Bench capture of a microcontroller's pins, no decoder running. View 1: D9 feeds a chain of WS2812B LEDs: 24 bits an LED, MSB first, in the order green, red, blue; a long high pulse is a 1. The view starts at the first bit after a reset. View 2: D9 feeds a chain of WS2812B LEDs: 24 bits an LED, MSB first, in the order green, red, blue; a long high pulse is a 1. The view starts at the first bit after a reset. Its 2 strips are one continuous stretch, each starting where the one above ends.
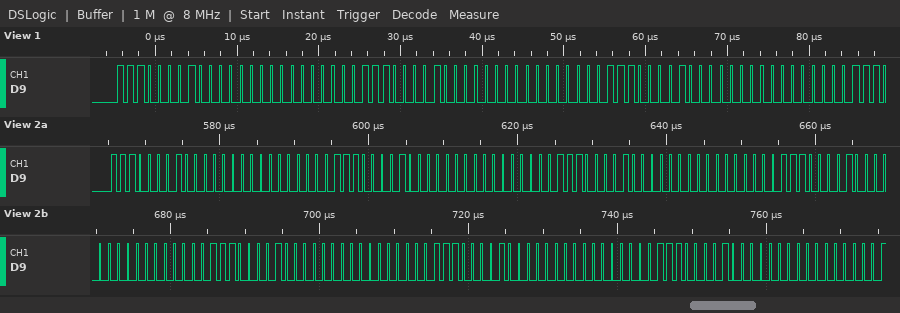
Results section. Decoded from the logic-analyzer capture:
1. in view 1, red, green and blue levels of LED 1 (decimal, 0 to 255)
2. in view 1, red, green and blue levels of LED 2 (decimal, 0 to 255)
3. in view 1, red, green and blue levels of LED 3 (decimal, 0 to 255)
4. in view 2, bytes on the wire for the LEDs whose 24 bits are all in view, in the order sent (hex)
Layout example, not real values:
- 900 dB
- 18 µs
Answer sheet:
- 0, 225, 0
- 0, 225, 0
- 0, 225, 0
- E1 00 00 E1 00 00 E1 00 00 E1 00 00 E1 00 00 E1 00 00 E1 00 00
